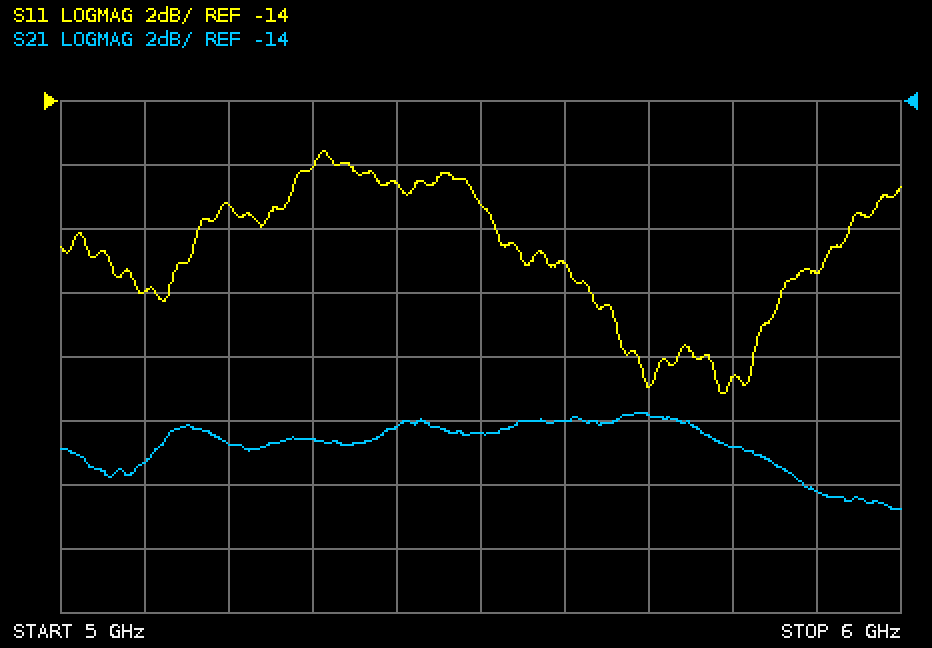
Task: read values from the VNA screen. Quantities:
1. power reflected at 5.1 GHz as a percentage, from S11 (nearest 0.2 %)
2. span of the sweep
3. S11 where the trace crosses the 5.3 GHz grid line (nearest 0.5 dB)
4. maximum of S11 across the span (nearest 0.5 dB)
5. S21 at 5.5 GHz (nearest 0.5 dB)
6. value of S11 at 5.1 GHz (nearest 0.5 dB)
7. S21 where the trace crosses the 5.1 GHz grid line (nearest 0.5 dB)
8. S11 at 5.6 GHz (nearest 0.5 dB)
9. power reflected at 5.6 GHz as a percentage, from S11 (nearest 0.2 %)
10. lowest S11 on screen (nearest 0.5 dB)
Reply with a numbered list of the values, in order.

1. 1.0 %
2. 1 GHz
3. -16.0 dB
4. -15.5 dB
5. -24.5 dB
6. -20.0 dB
7. -25.5 dB
8. -19.0 dB
9. 1.2 %
10. -23.0 dB
